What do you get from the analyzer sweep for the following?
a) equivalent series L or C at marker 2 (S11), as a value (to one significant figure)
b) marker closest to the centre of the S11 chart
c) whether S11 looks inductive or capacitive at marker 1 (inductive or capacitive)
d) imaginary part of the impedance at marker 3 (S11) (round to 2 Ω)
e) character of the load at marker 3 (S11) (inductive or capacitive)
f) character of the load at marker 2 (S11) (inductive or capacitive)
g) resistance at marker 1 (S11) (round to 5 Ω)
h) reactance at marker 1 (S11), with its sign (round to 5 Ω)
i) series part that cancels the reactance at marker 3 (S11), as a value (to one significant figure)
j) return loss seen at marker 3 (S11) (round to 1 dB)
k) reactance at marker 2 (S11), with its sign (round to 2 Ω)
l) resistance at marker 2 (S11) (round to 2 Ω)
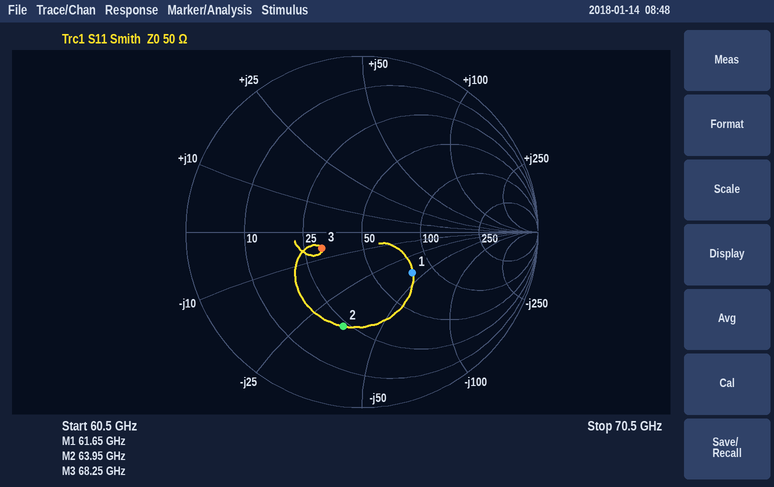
70 fF
marker 3
capacitive
-6 Ω
capacitive
capacitive
75 Ω
-40 Ω
10 pH
12 dB
-36 Ω
24 Ω
